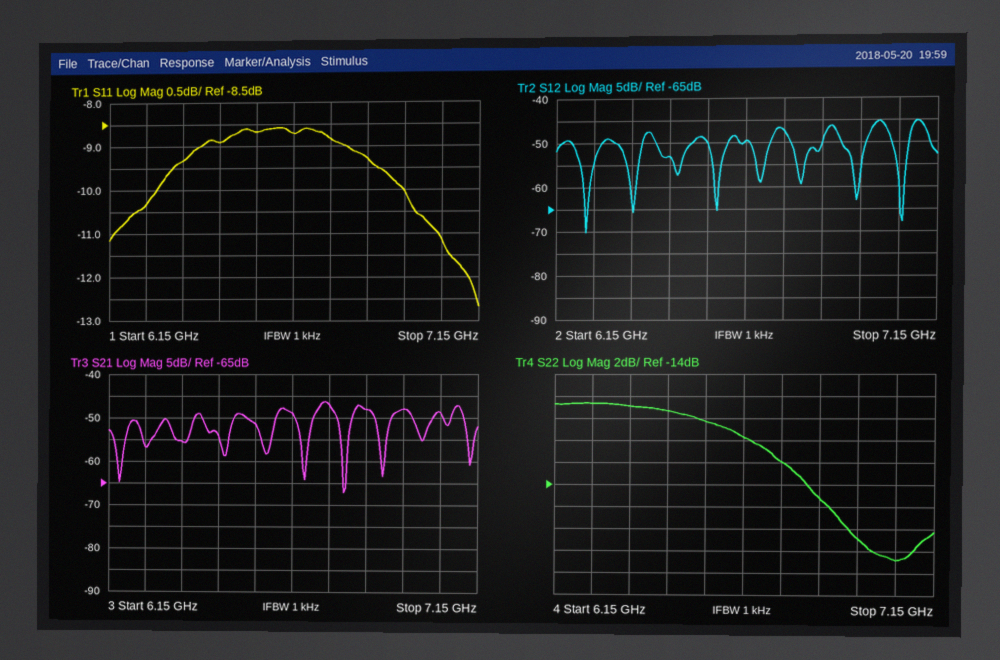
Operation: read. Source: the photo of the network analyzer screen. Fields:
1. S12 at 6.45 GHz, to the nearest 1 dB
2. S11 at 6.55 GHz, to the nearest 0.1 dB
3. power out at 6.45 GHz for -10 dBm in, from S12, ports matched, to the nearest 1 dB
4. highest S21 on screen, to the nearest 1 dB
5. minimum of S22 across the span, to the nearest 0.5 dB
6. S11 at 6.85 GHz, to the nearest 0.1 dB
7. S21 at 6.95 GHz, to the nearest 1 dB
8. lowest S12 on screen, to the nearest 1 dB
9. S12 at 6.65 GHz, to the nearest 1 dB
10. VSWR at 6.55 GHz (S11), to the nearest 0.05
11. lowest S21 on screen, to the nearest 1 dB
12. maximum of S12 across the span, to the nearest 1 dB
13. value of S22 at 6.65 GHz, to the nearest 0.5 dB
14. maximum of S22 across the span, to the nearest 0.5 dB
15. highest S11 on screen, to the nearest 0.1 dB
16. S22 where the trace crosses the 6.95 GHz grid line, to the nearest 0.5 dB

-53 dB
-8.7 dB
-63 dBm
-46 dB
-21.0 dB
-9.3 dB
-48 dB
-70 dB
-50 dB
2.15
-67 dB
-45 dB
-9.5 dB
-6.5 dB
-8.6 dB
-19.0 dB
